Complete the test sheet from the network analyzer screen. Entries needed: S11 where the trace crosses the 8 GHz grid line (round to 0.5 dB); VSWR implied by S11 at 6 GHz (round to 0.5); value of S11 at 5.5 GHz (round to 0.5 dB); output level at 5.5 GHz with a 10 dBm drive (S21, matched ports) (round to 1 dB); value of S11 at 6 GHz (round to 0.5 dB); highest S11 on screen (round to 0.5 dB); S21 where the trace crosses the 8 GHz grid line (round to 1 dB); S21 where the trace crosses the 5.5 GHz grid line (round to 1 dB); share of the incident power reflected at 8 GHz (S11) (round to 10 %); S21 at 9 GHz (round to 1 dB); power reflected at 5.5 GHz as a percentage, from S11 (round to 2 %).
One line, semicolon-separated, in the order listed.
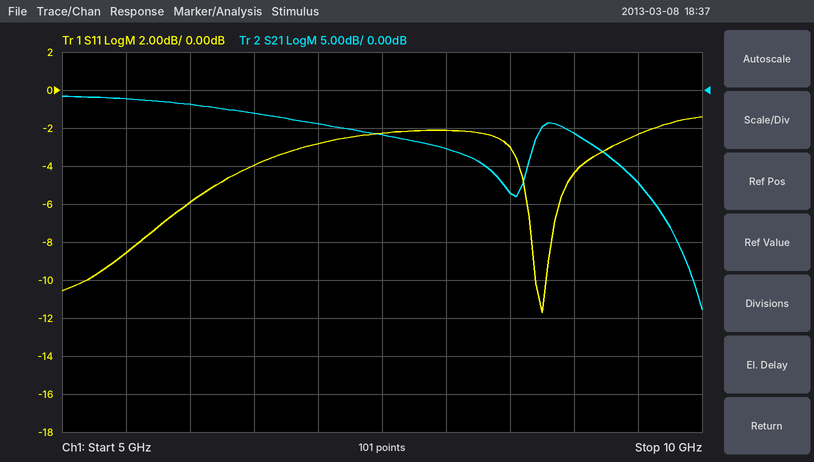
-2.0 dB; 3.0; -8.5 dB; 9 dBm; -6.0 dB; -1.5 dB; -8 dB; -1 dB; 60 %; -6 dB; 14 %
